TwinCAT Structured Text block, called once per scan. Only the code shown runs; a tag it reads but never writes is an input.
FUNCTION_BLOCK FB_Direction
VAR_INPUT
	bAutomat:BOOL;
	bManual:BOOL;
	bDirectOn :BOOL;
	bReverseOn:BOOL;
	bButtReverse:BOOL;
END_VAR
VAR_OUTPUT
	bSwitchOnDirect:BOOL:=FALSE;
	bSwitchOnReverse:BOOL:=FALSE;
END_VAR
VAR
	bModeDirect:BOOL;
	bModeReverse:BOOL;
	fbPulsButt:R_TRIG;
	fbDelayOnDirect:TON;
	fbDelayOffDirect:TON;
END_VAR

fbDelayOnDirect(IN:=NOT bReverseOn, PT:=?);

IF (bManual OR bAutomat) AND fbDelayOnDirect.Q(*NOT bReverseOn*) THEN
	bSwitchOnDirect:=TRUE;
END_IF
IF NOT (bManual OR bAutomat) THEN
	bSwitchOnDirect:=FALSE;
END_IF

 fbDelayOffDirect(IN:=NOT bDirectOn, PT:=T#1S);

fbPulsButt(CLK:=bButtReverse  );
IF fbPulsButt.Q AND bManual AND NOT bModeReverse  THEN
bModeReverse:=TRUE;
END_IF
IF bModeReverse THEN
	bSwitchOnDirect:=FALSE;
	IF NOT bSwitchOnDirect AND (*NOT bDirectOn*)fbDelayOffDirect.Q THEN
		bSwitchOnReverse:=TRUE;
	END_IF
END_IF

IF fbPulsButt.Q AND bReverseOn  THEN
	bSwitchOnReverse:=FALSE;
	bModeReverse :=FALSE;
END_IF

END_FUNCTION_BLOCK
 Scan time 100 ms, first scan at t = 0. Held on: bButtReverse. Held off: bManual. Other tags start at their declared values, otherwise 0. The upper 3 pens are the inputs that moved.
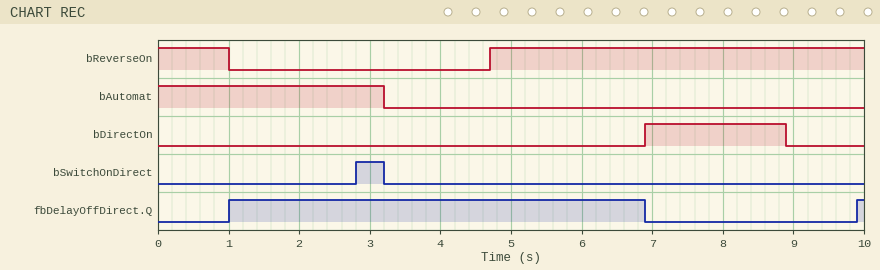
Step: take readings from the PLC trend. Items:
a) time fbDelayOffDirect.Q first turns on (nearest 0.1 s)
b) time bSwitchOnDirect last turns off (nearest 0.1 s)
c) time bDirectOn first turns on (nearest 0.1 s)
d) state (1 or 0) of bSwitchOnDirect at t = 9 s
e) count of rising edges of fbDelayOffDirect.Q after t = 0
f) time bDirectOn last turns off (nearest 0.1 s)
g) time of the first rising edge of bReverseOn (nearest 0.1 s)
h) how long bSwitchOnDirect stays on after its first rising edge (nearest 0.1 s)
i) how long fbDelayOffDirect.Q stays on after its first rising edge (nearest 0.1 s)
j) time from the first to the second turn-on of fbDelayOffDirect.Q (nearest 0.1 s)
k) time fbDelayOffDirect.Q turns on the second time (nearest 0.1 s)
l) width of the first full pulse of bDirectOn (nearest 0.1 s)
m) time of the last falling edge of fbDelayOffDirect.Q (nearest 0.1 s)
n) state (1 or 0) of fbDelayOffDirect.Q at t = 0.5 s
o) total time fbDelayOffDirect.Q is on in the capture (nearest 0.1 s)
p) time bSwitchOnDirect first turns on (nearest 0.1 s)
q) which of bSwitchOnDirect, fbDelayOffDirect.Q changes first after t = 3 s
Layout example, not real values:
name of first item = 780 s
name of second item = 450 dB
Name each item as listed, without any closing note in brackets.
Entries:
time fbDelayOffDirect.Q first turns on = 1.0 s
time bSwitchOnDirect last turns off = 3.2 s
time bDirectOn first turns on = 6.9 s
state (1 or 0) of bSwitchOnDirect at t = 9 s = 0
count of rising edges of fbDelayOffDirect.Q after t = 0 = 2
time bDirectOn last turns off = 8.9 s
time of the first rising edge of bReverseOn = 4.7 s
how long bSwitchOnDirect stays on after its first rising edge = 0.4 s
how long fbDelayOffDirect.Q stays on after its first rising edge = 5.9 s
time from the first to the second turn-on of fbDelayOffDirect.Q = 8.9 s
time fbDelayOffDirect.Q turns on the second time = 9.9 s
width of the first full pulse of bDirectOn = 2.0 s
time of the last falling edge of fbDelayOffDirect.Q = 6.9 s
state (1 or 0) of fbDelayOffDirect.Q at t = 0.5 s = 0
total time fbDelayOffDirect.Q is on in the capture = 6.0 s
time bSwitchOnDirect first turns on = 2.8 s
which of bSwitchOnDirect, fbDelayOffDirect.Q changes first after t = 3 s = bSwitchOnDirect
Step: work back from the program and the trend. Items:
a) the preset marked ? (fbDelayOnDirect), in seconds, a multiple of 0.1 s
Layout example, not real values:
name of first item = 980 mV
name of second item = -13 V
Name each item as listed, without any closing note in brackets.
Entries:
the preset marked ? (fbDelayOnDirect), in seconds, a multiple of 0.1 s = 1.8 s
